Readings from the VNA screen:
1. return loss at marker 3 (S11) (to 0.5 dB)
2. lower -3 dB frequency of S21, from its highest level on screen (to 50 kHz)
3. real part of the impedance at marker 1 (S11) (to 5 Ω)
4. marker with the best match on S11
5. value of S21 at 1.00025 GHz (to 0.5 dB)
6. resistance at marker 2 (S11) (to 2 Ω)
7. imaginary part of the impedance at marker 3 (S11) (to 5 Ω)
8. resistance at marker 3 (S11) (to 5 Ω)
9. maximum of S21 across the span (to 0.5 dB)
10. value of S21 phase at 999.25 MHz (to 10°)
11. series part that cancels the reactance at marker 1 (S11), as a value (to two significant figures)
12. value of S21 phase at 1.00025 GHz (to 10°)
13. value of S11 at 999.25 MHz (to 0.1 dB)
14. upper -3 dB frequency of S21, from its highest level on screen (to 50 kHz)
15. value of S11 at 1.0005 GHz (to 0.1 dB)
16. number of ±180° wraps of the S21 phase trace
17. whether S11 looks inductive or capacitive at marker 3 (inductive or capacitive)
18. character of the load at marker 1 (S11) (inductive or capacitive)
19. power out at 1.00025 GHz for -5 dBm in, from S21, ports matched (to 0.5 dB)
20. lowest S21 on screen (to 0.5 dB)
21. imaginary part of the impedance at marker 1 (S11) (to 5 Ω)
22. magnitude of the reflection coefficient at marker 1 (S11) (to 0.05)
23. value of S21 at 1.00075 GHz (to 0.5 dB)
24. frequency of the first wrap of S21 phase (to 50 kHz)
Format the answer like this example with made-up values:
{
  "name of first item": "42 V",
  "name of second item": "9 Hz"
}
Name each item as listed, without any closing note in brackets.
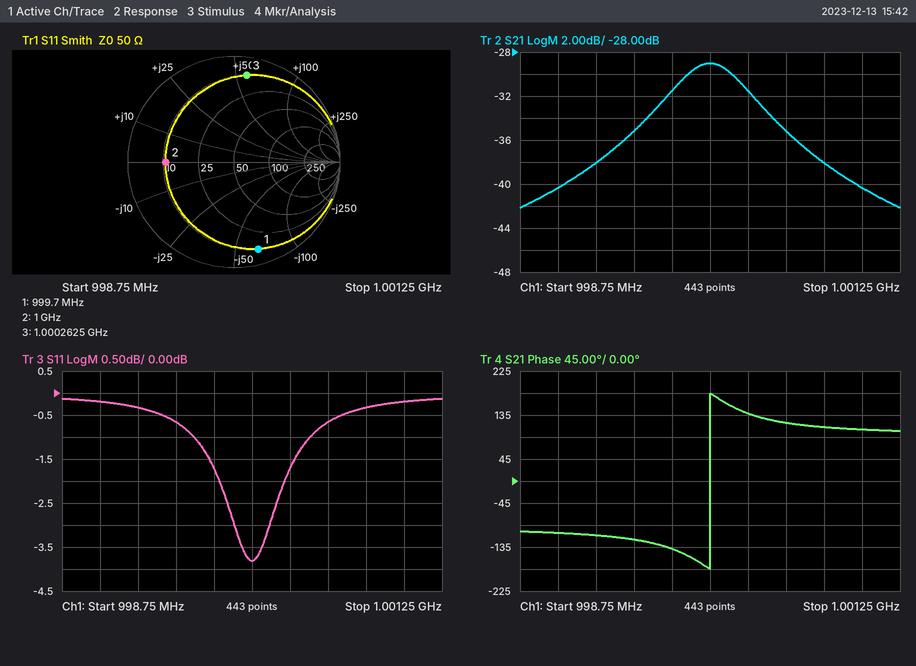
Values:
{
  "return loss at marker 3 (S11)": "1.5 dB",
  "lower -3 dB frequency of S21, from its highest level on screen": "999.70 MHz",
  "real part of the impedance at marker 1 (S11)": "10 Ω",
  "marker with the best match on S11": "marker 2",
  "value of S21 at 1.00025 GHz": "-31.5 dB",
  "resistance at marker 2 (S11)": "10 Ω",
  "imaginary part of the impedance at marker 3 (S11)": "+55 Ω",
  "resistance at marker 3 (S11)": "10 Ω",
  "maximum of S21 across the span": "-29.0 dB",
  "value of S21 phase at 999.25 MHz": "-110°",
  "series part that cancels the reactance at marker 1 (S11), as a value": "10 nH",
  "value of S21 phase at 1.00025 GHz": "140°",
  "value of S11 at 999.25 MHz": "-0.3 dB",
  "upper -3 dB frequency of S21, from its highest level on screen": "1.00030 GHz",
  "value of S11 at 1.0005 GHz": "-0.7 dB",
  "number of ±180° wraps of the S21 phase trace": "1",
  "whether S11 looks inductive or capacitive at marker 3": "inductive",
  "character of the load at marker 1 (S11)": "capacitive",
  "power out at 1.00025 GHz for -5 dBm in, from S21, ports matched": "-36.5 dBm",
  "lowest S21 on screen": "-42.0 dB",
  "imaginary part of the impedance at marker 1 (S11)": "-65 Ω",
  "magnitude of the reflection coefficient at marker 1 (S11)": "0.85",
  "value of S21 at 1.00075 GHz": "-38.0 dB",
  "frequency of the first wrap of S21 phase": "1.00000 GHz"
}
